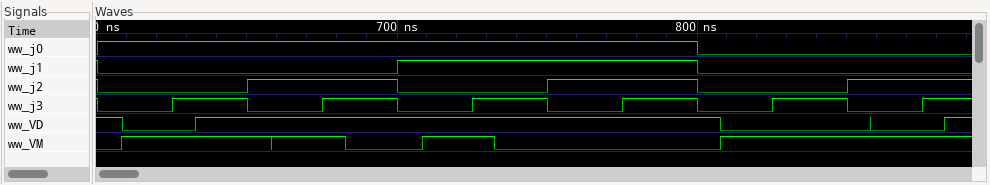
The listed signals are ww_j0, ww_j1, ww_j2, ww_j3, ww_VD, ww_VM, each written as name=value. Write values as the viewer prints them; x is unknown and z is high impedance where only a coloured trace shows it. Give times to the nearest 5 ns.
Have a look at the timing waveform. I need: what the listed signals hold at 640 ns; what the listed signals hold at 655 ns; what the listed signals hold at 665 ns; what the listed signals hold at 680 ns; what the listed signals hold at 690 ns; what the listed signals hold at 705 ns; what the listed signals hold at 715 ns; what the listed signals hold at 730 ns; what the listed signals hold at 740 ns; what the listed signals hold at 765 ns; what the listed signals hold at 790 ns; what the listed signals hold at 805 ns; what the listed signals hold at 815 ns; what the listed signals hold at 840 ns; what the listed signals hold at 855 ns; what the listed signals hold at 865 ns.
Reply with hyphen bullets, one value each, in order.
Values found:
- ww_j0=1, ww_j1=0, ww_j2=0, ww_j3=1, ww_VD=1, ww_VM=1
- ww_j0=1, ww_j1=0, ww_j2=1, ww_j3=0, ww_VD=1, ww_VM=1
- ww_j0=1, ww_j1=0, ww_j2=1, ww_j3=0, ww_VD=1, ww_VM=1
- ww_j0=1, ww_j1=0, ww_j2=1, ww_j3=1, ww_VD=1, ww_VM=1
- ww_j0=1, ww_j1=0, ww_j2=1, ww_j3=1, ww_VD=1, ww_VM=0
- ww_j0=1, ww_j1=1, ww_j2=0, ww_j3=0, ww_VD=1, ww_VM=0
- ww_j0=1, ww_j1=1, ww_j2=0, ww_j3=0, ww_VD=1, ww_VM=1
- ww_j0=1, ww_j1=1, ww_j2=0, ww_j3=1, ww_VD=1, ww_VM=1
- ww_j0=1, ww_j1=1, ww_j2=0, ww_j3=1, ww_VD=1, ww_VM=0
- ww_j0=1, ww_j1=1, ww_j2=1, ww_j3=0, ww_VD=1, ww_VM=0
- ww_j0=1, ww_j1=1, ww_j2=1, ww_j3=1, ww_VD=1, ww_VM=0
- ww_j0=0, ww_j1=0, ww_j2=0, ww_j3=0, ww_VD=1, ww_VM=0
- ww_j0=0, ww_j1=0, ww_j2=0, ww_j3=0, ww_VD=0, ww_VM=1
- ww_j0=0, ww_j1=0, ww_j2=0, ww_j3=1, ww_VD=0, ww_VM=1
- ww_j0=0, ww_j1=0, ww_j2=1, ww_j3=0, ww_VD=0, ww_VM=1
- ww_j0=0, ww_j1=0, ww_j2=1, ww_j3=0, ww_VD=0, ww_VM=1
